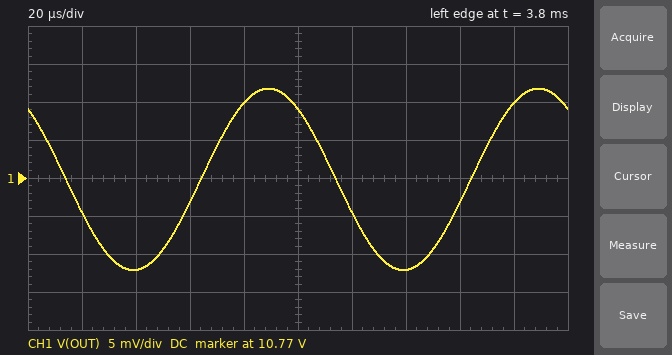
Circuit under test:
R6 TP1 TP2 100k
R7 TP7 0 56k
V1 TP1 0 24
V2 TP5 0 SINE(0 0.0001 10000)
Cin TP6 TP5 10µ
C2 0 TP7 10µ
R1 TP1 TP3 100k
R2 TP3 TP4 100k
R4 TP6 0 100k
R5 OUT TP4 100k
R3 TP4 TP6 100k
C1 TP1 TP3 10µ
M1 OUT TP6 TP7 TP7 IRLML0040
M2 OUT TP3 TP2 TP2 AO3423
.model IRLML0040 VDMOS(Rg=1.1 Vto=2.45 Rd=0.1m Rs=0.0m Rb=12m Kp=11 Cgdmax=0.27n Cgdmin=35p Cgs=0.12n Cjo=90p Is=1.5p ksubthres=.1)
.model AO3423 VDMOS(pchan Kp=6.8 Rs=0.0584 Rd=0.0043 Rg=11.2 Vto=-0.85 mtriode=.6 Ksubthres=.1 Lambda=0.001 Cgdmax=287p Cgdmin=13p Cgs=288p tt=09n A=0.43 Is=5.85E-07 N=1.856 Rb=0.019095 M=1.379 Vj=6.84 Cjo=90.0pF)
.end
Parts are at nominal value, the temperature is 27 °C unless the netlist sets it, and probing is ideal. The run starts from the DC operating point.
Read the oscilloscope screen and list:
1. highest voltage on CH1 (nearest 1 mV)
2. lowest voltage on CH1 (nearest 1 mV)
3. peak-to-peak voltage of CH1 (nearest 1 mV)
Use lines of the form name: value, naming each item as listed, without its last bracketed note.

highest voltage on CH1: 10.782 V
lowest voltage on CH1: 10.758 V
peak-to-peak voltage of CH1: 24 mV
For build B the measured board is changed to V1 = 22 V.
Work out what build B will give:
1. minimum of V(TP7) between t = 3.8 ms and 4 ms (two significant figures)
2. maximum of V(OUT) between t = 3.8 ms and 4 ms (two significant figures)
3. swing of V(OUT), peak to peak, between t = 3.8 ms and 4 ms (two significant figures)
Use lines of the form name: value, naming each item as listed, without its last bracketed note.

minimum of V(TP7) between t = 3.8 ms and 4 ms: 3.2 V
maximum of V(OUT) between t = 3.8 ms and 4 ms: 10 V
swing of V(OUT), peak to peak, between t = 3.8 ms and 4 ms: 21 mV
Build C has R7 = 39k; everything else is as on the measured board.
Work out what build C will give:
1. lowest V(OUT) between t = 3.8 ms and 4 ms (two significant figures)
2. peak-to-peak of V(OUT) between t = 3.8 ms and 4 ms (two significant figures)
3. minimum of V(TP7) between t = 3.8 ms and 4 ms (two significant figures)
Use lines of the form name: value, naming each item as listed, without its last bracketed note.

lowest V(OUT) between t = 3.8 ms and 4 ms: 8.8 V
peak-to-peak of V(OUT) between t = 3.8 ms and 4 ms: 29 mV
minimum of V(TP7) between t = 3.8 ms and 4 ms: 3.1 V
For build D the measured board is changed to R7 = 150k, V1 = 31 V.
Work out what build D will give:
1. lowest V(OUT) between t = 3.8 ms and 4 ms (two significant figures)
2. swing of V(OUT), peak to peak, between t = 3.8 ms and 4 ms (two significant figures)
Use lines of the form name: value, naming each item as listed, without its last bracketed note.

lowest V(OUT) between t = 3.8 ms and 4 ms: 19 V
swing of V(OUT), peak to peak, between t = 3.8 ms and 4 ms: 17 mV
